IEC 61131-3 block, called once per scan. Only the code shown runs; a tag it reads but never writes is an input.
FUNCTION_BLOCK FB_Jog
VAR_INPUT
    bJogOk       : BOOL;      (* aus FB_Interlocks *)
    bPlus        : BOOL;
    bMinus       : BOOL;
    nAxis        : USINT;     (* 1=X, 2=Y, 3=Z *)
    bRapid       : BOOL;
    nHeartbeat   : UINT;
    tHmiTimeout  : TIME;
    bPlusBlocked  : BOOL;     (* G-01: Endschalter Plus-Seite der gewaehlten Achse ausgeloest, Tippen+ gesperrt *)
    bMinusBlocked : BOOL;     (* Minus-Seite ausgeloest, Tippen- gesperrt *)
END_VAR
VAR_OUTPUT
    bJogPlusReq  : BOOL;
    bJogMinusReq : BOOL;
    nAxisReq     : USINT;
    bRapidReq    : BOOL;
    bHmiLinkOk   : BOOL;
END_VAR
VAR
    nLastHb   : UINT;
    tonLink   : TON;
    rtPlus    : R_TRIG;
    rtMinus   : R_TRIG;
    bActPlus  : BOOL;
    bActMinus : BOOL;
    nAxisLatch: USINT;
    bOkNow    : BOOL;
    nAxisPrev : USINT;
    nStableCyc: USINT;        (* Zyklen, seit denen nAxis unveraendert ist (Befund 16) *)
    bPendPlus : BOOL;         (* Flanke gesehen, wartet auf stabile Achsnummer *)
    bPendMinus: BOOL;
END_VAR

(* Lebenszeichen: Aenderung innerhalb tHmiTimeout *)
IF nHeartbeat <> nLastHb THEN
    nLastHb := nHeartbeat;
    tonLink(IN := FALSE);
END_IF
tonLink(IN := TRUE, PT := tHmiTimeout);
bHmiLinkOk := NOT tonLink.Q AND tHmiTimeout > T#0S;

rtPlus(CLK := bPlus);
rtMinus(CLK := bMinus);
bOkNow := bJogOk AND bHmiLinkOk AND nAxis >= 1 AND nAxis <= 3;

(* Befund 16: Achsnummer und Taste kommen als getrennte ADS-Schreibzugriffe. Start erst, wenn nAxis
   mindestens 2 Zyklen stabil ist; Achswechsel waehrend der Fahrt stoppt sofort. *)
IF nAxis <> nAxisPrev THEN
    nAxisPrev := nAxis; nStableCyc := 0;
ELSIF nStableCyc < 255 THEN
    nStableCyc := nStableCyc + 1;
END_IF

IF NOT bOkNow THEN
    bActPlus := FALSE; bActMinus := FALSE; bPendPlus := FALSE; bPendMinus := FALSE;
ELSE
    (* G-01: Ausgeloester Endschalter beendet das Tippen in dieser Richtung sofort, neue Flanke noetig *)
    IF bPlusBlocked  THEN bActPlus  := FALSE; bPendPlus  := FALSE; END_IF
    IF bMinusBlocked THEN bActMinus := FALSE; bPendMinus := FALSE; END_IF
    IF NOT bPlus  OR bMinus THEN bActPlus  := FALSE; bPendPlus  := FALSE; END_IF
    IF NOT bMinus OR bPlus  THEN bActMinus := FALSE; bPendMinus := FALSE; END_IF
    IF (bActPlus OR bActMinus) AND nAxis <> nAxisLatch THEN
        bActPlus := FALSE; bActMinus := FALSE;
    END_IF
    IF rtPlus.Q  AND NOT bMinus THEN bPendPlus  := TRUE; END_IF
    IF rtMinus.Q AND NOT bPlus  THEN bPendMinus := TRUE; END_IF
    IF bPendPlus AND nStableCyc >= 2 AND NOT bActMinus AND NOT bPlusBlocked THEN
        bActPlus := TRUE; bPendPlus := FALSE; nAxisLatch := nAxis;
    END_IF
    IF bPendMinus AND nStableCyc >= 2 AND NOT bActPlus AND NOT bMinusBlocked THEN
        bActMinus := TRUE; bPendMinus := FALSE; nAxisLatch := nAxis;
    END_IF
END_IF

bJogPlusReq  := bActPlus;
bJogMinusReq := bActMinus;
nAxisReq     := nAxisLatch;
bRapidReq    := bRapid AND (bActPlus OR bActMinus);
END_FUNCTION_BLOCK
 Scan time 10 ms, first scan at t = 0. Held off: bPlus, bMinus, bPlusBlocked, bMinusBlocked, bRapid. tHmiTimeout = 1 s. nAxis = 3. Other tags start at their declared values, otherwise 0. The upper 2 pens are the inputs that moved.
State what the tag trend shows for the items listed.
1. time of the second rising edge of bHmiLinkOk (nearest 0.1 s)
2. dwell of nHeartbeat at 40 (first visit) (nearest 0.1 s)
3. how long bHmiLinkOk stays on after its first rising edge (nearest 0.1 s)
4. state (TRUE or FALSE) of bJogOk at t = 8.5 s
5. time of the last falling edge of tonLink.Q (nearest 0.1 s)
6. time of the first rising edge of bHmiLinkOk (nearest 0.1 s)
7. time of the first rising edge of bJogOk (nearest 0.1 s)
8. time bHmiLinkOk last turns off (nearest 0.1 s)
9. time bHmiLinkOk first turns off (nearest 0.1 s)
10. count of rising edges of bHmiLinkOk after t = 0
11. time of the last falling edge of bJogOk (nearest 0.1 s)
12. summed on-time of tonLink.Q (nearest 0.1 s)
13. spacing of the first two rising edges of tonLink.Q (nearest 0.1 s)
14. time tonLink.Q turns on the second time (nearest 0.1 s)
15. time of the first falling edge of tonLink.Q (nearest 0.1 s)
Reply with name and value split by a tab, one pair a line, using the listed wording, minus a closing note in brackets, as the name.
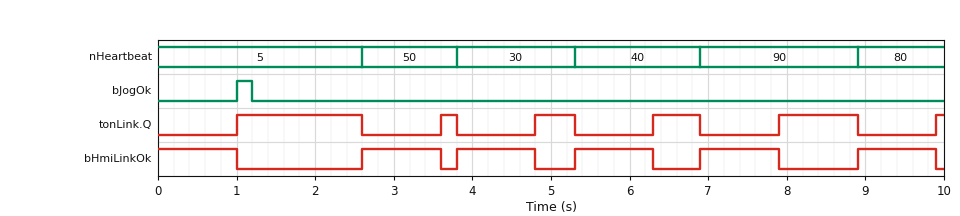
time of the second rising edge of bHmiLinkOk	3.8 s
dwell of nHeartbeat at 40 (first visit)	1.6 s
how long bHmiLinkOk stays on after its first rising edge	1.0 s
state (TRUE or FALSE) of bJogOk at t = 8.5 s	FALSE
time of the last falling edge of tonLink.Q	8.9 s
time of the first rising edge of bHmiLinkOk	2.6 s
time of the first rising edge of bJogOk	1.0 s
time bHmiLinkOk last turns off	9.9 s
time bHmiLinkOk first turns off	1.0 s
count of rising edges of bHmiLinkOk after t = 0	5
time of the last falling edge of bJogOk	1.2 s
summed on-time of tonLink.Q	4.0 s
spacing of the first two rising edges of tonLink.Q	2.6 s
time tonLink.Q turns on the second time	3.6 s
time of the first falling edge of tonLink.Q	2.6 s
